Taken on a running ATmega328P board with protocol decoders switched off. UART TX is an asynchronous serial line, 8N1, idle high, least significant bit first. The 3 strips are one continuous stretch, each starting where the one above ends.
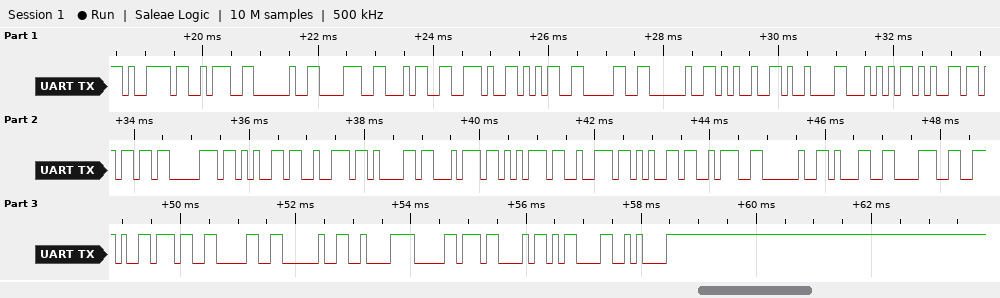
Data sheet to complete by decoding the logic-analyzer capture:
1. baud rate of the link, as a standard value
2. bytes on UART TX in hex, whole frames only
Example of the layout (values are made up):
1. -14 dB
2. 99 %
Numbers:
1. 9600 baud
2. 79 3A 20 38 34 2E 35 30 20 25 09 54 65 6D 70 65 72 61 74 75 72 65 3A 20 31 38 2E 37 30 20 C2 B0 43 0D 0A
